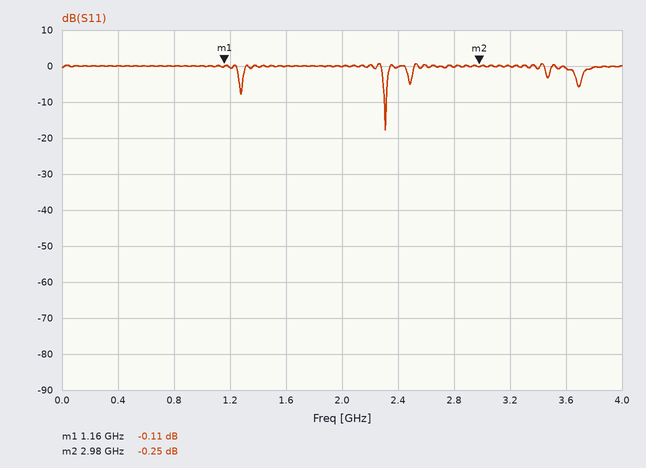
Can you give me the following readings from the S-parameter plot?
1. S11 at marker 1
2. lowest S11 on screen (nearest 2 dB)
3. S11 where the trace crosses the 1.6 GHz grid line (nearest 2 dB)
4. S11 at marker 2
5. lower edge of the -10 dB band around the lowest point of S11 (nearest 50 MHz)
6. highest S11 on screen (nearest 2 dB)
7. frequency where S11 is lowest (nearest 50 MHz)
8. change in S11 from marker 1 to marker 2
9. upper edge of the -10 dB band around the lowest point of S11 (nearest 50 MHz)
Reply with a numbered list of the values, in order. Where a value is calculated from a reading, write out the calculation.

1. -0.11 dB
2. -18 dB
3. 0 dB
4. -0.25 dB
5. 2.30 GHz
6. 0 dB
7. 2.30 GHz
8. -0.25 − (-0.11) = -0.14 dB
9. 2.30 GHz
